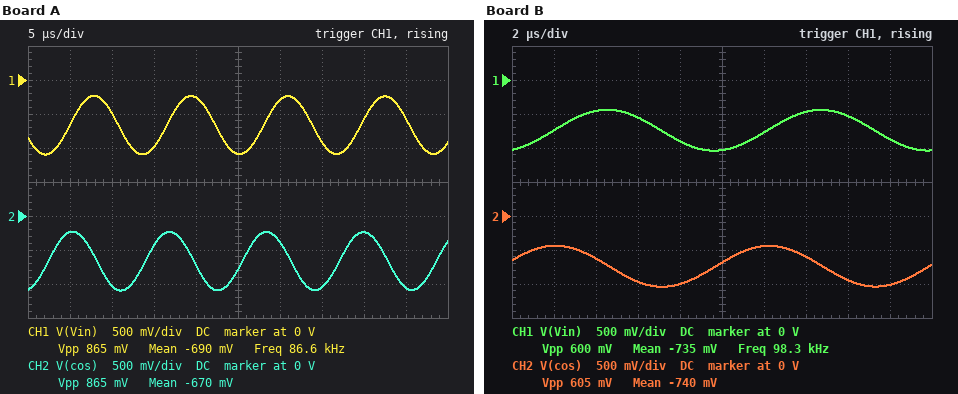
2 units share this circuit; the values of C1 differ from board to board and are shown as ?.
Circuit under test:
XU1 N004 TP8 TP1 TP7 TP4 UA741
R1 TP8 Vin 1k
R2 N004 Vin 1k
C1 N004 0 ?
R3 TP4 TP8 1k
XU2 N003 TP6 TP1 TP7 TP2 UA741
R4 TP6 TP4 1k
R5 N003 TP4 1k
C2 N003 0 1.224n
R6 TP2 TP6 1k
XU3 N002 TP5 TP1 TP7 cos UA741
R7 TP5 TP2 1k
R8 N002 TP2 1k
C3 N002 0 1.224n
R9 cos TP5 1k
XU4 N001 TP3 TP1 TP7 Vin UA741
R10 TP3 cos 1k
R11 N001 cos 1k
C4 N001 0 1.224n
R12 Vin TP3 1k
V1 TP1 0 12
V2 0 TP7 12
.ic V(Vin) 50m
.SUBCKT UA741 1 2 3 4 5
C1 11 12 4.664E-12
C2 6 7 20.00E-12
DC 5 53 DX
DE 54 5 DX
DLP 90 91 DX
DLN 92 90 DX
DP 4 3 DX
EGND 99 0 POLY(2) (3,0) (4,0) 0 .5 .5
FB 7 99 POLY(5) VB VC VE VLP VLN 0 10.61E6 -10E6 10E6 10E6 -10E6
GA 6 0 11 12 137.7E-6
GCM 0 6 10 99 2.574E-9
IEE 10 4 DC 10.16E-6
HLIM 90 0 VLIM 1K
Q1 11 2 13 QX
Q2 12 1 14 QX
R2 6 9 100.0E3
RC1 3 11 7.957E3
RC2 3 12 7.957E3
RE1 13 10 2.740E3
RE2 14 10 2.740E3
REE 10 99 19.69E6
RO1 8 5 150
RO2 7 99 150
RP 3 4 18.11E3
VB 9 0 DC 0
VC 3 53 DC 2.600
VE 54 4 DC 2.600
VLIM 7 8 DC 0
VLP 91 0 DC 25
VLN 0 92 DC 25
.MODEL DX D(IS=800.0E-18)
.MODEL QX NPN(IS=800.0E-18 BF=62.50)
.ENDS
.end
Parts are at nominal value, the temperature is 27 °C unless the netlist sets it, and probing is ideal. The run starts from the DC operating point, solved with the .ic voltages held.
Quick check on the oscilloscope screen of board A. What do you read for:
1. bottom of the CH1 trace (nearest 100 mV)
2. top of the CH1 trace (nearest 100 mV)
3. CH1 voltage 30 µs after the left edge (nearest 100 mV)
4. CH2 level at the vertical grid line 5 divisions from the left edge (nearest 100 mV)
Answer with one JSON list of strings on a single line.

["-1.1 V", "-200 mV", "-300 mV", "-800 mV"]
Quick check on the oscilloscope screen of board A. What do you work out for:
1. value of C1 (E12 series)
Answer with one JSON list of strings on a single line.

["2.7 nF"]
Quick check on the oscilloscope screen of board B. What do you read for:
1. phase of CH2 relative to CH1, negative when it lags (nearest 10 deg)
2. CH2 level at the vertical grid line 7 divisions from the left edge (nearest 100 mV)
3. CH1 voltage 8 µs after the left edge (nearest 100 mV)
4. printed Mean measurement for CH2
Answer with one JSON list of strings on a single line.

["90 deg", "-600 mV", "-900 mV", "-740 mV"]
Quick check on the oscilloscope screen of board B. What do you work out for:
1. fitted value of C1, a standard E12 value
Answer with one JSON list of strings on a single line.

["1.5 nF"]
